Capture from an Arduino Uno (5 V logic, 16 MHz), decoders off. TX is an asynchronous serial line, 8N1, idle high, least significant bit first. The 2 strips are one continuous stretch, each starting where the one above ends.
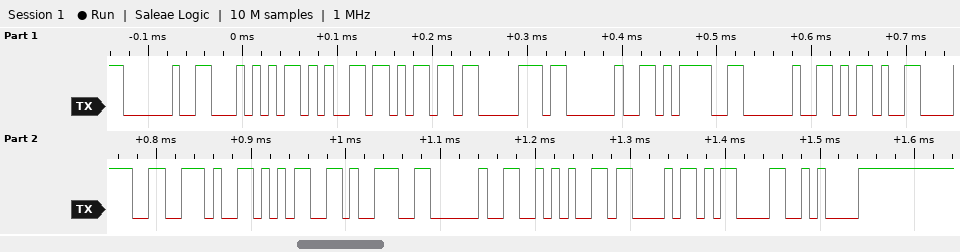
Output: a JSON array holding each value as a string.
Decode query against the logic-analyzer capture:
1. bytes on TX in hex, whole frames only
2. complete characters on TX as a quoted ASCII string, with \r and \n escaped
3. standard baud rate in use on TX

["20 54 65 6D 70 20 3D 20 2D 38 2E 35 39 20 2A 43 0D 0A", "\" Temp = -8.59 *C\\r\\n\"", "115200 baud"]
